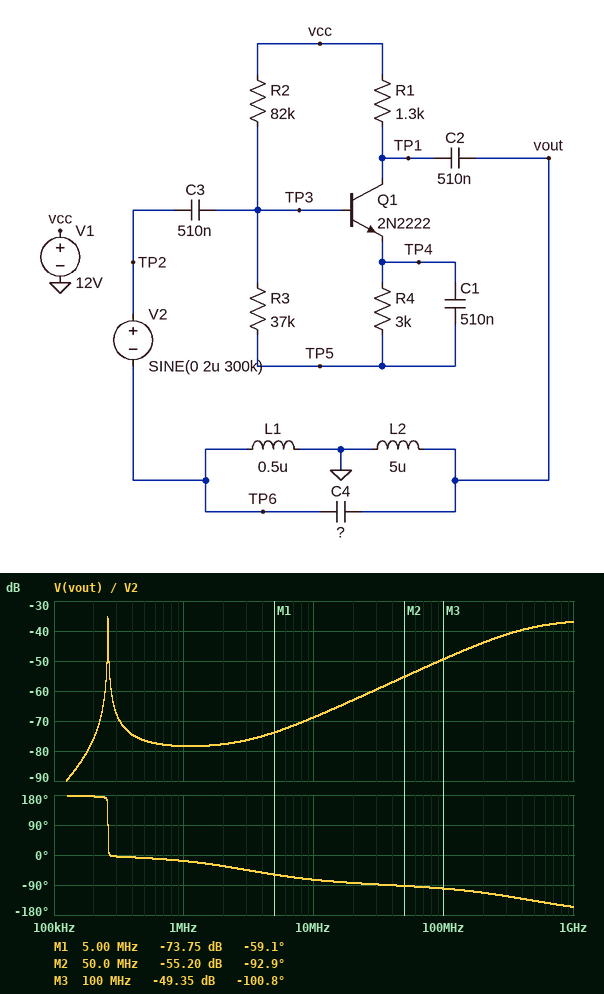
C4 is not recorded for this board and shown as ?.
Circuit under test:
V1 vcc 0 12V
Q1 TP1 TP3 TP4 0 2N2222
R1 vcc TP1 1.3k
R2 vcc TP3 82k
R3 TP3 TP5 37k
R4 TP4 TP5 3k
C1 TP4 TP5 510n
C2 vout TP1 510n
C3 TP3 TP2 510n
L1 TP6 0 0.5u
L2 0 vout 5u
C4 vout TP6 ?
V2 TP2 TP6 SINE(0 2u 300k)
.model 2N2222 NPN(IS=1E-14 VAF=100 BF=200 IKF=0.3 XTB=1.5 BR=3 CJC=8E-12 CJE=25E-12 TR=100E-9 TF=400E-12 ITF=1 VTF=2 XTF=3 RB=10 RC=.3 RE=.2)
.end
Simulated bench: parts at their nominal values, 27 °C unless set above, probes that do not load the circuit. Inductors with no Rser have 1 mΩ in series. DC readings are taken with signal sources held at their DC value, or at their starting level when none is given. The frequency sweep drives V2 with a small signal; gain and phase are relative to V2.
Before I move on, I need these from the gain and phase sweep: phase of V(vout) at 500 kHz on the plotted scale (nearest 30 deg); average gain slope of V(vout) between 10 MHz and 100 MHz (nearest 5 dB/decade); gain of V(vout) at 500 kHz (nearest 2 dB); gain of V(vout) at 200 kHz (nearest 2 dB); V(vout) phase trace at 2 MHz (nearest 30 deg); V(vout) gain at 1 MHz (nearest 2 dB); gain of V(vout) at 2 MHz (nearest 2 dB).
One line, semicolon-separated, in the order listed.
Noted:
0 deg; 20 dB/decade; -76 dB; -76 dB; -30 deg; -78 dB; -78 dB
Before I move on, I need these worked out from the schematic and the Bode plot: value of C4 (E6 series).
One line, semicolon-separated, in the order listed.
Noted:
68 nF
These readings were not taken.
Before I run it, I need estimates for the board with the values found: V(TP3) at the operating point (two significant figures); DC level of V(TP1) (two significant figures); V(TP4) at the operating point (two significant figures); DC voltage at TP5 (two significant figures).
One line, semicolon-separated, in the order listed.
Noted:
12 V; 12 V; 12 V; 12 V
